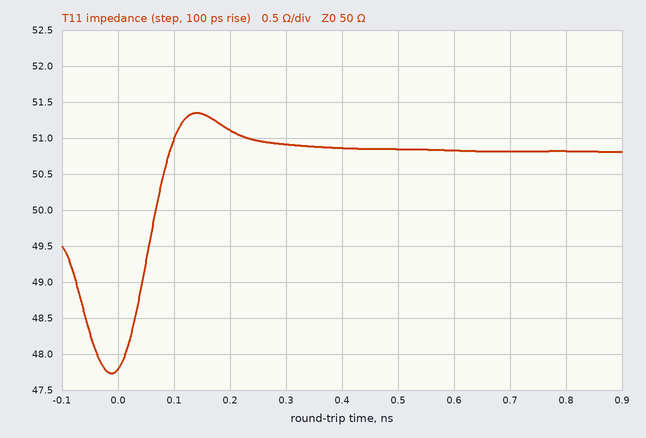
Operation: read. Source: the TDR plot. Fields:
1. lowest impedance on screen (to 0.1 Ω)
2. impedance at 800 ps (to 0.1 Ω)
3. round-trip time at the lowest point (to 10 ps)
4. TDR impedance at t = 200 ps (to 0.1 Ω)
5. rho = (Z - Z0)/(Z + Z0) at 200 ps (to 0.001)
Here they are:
47.7 Ω
50.8 Ω
-10 ps
51.1 Ω
+0.011
